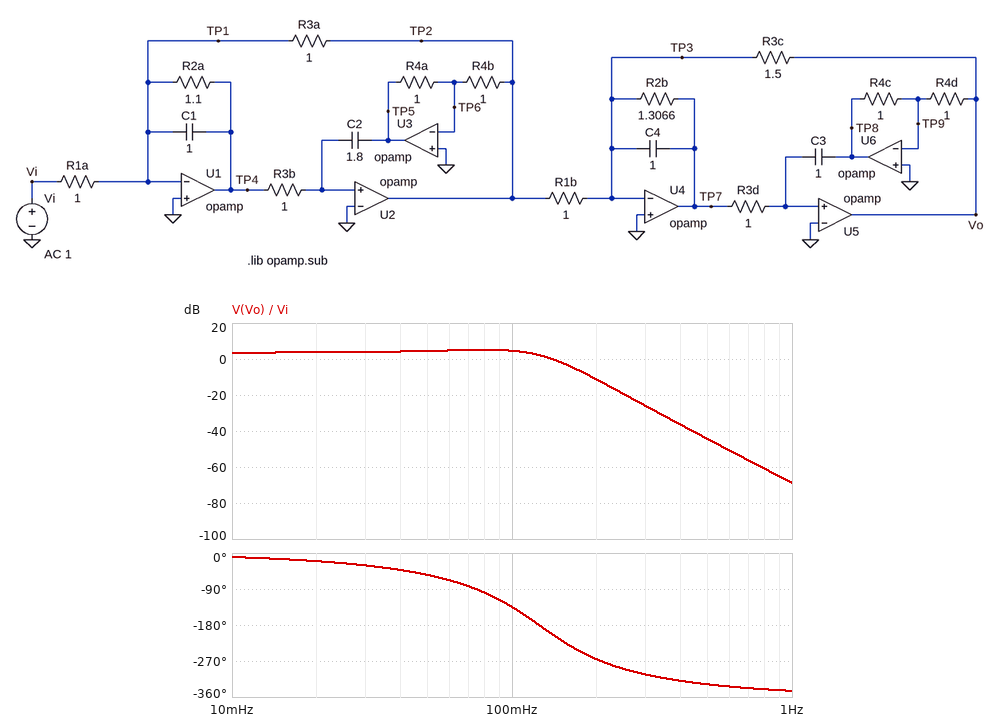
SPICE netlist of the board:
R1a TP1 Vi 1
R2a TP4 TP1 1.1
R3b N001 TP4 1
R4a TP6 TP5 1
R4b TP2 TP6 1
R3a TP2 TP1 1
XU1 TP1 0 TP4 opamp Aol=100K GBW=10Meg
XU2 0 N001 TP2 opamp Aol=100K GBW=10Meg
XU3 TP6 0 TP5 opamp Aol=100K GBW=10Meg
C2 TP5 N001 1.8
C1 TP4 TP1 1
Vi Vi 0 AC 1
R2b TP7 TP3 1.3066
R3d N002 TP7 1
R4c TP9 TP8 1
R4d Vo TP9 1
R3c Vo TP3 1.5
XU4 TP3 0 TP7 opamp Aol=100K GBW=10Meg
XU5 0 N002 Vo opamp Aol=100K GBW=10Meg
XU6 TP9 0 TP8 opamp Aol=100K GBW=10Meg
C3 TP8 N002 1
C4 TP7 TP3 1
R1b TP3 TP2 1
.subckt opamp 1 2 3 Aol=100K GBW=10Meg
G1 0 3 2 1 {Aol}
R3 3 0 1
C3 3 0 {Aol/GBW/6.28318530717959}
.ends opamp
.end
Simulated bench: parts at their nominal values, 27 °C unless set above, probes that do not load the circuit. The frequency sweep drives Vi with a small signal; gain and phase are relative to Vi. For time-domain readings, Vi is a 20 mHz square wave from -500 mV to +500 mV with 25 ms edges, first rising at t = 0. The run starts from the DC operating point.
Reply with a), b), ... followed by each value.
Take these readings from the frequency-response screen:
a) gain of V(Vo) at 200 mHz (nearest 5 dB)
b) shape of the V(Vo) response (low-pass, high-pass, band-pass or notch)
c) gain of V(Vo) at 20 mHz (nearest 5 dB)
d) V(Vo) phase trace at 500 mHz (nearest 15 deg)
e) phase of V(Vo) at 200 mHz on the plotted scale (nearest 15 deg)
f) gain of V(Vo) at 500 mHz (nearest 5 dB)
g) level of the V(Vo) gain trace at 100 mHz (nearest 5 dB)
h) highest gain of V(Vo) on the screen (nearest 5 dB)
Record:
a) -10 dB
b) low-pass
c) 5 dB
d) -330 deg
e) -270 deg
f) -45 dB
g) 5 dB
h) 5 dB
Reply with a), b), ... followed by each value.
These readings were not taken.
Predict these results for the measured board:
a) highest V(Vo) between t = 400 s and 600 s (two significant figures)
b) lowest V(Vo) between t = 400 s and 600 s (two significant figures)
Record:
a) 1.1 V
b) -1.1 V
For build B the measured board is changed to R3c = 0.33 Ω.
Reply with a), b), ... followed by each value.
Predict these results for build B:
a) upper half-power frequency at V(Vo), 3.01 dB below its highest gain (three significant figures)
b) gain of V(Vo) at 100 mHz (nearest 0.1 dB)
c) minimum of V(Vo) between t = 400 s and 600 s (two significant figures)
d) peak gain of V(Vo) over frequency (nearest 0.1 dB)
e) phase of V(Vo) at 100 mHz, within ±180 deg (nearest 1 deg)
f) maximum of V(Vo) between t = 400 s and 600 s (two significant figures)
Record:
a) 157 mHz
b) -9.1 dB
c) -200 mV
d) -8.8 dB
e) -85 deg
f) 200 mV
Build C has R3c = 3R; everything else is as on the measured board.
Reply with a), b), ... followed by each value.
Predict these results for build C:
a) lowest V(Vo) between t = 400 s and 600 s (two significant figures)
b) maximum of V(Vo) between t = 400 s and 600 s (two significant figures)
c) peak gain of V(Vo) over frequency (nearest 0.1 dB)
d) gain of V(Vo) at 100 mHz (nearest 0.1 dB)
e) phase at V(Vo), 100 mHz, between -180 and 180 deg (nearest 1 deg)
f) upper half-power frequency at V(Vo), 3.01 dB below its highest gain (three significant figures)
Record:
a) -1.8 V
b) 1.8 V
c) 9.8 dB
d) 5.7 dB
e) -172 deg
f) 92.6 mHz
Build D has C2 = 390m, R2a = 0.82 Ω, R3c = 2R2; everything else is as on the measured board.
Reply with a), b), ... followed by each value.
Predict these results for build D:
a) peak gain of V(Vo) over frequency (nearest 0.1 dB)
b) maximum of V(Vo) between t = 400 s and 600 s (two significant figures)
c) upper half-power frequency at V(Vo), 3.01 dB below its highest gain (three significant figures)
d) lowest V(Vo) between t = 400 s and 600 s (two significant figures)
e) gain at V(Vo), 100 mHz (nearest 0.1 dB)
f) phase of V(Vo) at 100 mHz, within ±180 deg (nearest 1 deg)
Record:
a) 7.9 dB
b) 1.4 V
c) 134 mHz
d) -1.4 V
e) 7.2 dB
f) -102 deg
